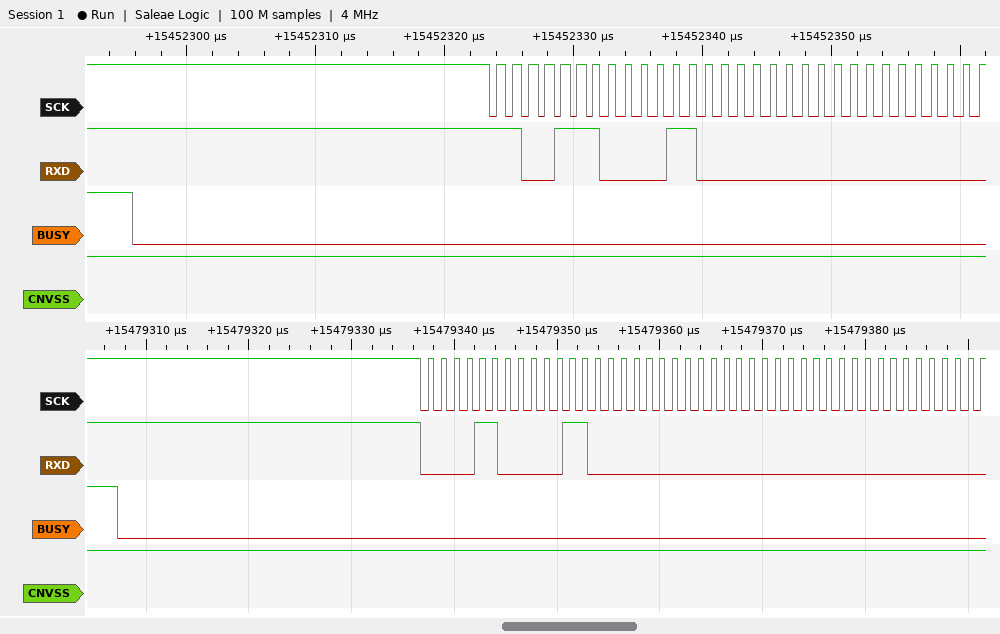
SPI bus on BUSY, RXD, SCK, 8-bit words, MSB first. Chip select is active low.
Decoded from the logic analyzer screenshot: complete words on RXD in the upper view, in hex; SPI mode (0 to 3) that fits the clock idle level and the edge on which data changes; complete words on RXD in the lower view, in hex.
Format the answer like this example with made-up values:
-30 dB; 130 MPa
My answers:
CE, 18, 00; 3; 0C, 18, 00, 00, 00
